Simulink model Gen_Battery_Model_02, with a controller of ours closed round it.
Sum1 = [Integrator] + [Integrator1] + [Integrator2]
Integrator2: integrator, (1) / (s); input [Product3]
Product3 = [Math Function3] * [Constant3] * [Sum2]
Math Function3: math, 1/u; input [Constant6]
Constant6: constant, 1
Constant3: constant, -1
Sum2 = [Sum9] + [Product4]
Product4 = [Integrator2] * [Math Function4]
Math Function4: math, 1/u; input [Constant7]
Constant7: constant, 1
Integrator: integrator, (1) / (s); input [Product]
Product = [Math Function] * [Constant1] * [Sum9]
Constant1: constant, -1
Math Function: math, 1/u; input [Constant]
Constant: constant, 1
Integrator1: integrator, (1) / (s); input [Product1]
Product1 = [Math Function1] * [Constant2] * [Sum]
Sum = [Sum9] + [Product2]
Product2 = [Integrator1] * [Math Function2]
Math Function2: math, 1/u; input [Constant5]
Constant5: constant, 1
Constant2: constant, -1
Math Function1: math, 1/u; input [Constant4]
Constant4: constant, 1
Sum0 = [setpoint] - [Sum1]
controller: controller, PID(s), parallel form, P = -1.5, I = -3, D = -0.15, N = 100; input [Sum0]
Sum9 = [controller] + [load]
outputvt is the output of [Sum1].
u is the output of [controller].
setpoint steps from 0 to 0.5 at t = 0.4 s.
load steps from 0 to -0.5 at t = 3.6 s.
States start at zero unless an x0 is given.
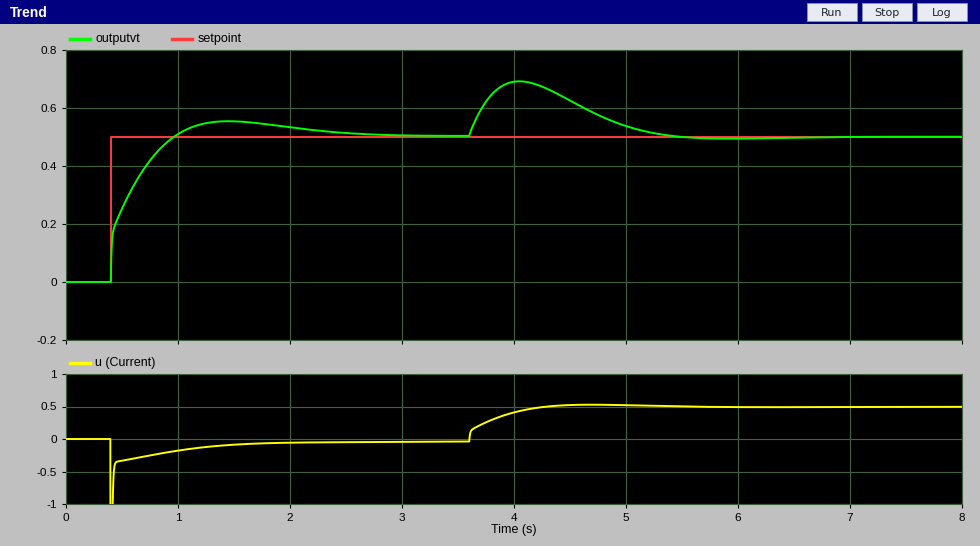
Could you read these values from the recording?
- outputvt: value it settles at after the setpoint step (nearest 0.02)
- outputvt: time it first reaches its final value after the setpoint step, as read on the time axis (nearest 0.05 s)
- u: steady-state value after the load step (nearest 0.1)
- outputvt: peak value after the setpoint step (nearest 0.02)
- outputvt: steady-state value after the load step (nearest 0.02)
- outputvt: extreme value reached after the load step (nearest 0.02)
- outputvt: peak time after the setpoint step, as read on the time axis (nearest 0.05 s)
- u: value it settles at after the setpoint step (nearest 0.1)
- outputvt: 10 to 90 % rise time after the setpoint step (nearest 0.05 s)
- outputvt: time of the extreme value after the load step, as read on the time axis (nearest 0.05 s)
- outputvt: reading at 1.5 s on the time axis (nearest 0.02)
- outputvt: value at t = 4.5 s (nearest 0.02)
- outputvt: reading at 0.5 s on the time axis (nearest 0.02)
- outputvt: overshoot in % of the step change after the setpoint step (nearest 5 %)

0.50
0.95 s
0.5
0.56
0.50
0.70
1.45 s
0.0
0.40 s
4.05 s
0.56
0.62
0.26
10 %
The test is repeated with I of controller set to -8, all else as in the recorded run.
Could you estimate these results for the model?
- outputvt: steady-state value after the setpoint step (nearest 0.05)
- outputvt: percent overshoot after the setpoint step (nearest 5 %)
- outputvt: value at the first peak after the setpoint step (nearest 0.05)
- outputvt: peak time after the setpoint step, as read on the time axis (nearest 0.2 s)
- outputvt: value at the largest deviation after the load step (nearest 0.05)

0.50
20 %
0.60
1.0 s
0.65
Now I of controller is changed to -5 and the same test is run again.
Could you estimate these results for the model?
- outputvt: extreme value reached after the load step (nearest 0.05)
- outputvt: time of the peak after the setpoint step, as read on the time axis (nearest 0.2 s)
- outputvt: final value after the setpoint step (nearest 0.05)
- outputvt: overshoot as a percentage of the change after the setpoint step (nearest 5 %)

0.65
1.2 s
0.50
15 %
